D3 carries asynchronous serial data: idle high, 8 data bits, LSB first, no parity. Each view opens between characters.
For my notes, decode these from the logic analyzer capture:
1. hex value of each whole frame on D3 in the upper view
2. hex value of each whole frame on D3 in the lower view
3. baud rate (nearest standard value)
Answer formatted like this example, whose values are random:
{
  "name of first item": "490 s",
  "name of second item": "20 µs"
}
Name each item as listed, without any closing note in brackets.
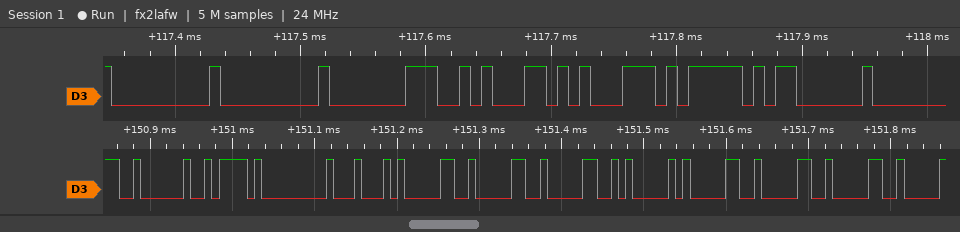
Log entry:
{
  "hex value of each whole frame on D3 in the upper view": "00, 00, C0, 8A, C5, 7D, 03",
  "hex value of each whole frame on D3 in the lower view": "02, 7A, 00, 44, 30, 30, 30, 41, 30, 30, 30",
  "baud rate": "115200 baud"
}
